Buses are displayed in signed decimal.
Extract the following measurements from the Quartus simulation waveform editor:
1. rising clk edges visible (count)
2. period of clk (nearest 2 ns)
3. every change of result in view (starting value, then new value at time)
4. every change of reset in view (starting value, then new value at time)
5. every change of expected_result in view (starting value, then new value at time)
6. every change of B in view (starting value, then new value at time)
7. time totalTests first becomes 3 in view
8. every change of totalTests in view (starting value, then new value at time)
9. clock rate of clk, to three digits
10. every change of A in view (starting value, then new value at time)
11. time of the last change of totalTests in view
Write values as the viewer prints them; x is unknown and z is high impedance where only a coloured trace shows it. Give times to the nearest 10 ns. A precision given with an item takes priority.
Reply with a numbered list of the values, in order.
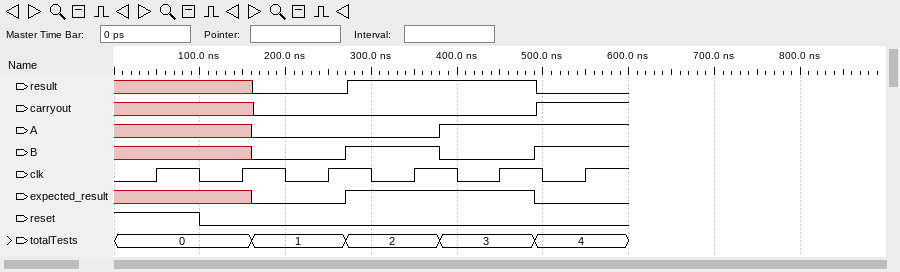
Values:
1. 6
2. 100 ns
3. x, 0 at 160 ns, 1 at 270 ns, 0 at 490 ns
4. 1, 0 at 100 ns
5. x, 0 at 160 ns, 1 at 270 ns, 0 at 490 ns
6. x, 0 at 160 ns, 1 at 270 ns, 0 at 380 ns, 1 at 490 ns
7. 380 ns
8. 0, 1 at 160 ns, 2 at 270 ns, 3 at 380 ns, 4 at 490 ns
9. 10.0 MHz
10. x, 0 at 160 ns, 1 at 380 ns
11. 490 ns
